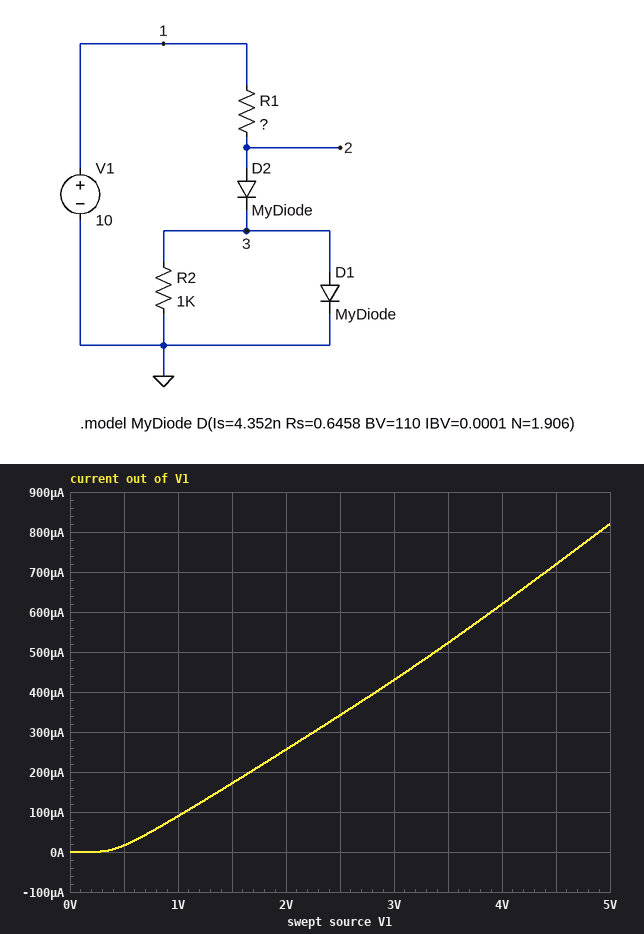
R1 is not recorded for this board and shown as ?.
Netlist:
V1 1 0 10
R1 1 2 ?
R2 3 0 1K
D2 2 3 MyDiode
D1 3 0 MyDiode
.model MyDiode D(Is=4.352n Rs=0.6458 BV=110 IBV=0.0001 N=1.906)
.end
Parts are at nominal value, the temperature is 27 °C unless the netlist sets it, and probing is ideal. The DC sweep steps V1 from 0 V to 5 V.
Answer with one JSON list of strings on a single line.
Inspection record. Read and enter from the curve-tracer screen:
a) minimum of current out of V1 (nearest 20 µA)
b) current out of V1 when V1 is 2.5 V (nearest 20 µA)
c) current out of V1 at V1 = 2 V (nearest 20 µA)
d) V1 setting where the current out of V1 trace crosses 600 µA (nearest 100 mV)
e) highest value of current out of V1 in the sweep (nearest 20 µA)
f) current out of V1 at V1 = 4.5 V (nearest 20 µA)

["0 A", "340 µA", "260 µA", "3.9 V", "820 µA", "720 µA"]
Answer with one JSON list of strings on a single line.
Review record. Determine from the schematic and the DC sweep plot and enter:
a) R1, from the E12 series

["4.7 kΩ"]
